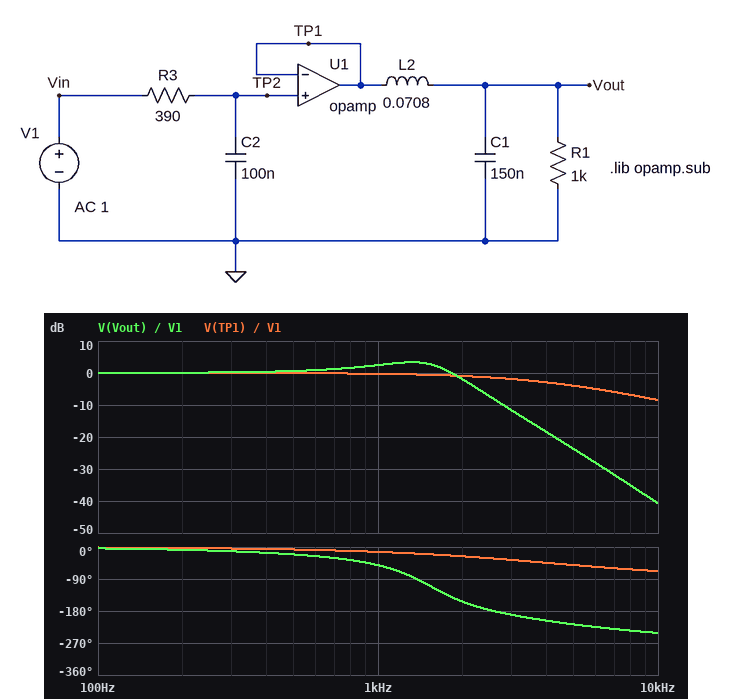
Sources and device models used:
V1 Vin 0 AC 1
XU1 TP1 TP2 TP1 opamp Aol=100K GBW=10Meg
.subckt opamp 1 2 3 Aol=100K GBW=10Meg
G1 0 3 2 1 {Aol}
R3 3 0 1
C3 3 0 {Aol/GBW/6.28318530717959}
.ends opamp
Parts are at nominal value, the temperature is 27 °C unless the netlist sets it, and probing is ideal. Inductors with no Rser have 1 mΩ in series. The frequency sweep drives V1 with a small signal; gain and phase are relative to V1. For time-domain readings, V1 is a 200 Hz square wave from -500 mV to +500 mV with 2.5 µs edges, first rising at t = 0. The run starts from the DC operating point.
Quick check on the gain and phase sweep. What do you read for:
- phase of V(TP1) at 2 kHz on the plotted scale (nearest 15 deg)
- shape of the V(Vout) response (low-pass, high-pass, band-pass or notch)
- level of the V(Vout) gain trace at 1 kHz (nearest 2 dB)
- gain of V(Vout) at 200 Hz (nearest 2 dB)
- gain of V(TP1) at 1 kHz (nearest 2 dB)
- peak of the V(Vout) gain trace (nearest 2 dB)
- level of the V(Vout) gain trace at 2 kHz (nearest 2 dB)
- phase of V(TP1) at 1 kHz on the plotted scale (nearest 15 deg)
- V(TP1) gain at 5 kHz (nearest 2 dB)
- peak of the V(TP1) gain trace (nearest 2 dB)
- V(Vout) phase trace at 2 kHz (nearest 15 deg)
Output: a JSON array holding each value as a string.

["-30 deg", "low-pass", "2 dB", "0 dB", "0 dB", "4 dB", "-2 dB", "-15 deg", "-4 dB", "0 dB", "-150 deg"]
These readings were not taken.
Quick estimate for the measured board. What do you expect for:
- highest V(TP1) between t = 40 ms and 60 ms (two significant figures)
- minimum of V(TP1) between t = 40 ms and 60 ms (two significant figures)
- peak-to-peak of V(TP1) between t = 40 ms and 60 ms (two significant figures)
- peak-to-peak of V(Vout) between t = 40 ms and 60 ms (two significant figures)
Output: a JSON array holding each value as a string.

["500 mV", "-500 mV", "1.0 V", "1.6 V"]
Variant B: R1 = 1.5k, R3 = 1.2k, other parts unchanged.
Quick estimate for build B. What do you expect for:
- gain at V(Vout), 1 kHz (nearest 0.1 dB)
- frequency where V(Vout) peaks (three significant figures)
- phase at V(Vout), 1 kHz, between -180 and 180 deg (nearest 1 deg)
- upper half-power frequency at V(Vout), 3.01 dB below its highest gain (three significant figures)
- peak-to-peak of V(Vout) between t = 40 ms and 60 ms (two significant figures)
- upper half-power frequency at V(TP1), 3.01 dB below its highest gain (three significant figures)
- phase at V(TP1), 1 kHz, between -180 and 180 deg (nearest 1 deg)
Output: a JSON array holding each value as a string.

["1.8 dB", "1.41 kHz", "-64 deg", "1.72 kHz", "1.5 V", "1.33 kHz", "-37 deg"]
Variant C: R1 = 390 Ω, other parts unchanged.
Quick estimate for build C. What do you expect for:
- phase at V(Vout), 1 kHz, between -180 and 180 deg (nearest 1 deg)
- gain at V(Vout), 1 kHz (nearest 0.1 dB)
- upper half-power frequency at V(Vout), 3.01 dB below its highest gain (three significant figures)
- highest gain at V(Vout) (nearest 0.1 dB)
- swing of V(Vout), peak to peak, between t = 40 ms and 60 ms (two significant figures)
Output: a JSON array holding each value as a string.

["-77 deg", "-2.4 dB", "1.12 kHz", "0 dB", "1.0 V"]
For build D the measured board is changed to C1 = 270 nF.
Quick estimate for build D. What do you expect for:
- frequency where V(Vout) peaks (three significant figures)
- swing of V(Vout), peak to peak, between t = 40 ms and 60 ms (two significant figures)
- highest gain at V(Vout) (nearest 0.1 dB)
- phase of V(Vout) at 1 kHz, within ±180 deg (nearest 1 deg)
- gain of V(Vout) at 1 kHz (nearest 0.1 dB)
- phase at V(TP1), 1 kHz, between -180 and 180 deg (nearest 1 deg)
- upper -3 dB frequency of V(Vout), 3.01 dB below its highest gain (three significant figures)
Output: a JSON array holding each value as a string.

["1.07 kHz", "1.8 V", "5.8 dB", "-75 deg", "5.6 dB", "-14 deg", "1.34 kHz"]
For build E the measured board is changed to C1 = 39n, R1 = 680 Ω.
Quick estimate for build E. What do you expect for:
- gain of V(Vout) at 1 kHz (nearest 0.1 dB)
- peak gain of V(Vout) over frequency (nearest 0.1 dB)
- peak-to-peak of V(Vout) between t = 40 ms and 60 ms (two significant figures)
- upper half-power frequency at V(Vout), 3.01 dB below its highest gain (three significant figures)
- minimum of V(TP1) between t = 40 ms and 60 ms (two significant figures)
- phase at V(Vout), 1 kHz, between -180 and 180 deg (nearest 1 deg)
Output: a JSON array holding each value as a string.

["-1.1 dB", "0 dB", "1.0 V", "1.70 kHz", "-500 mV", "-50 deg"]
